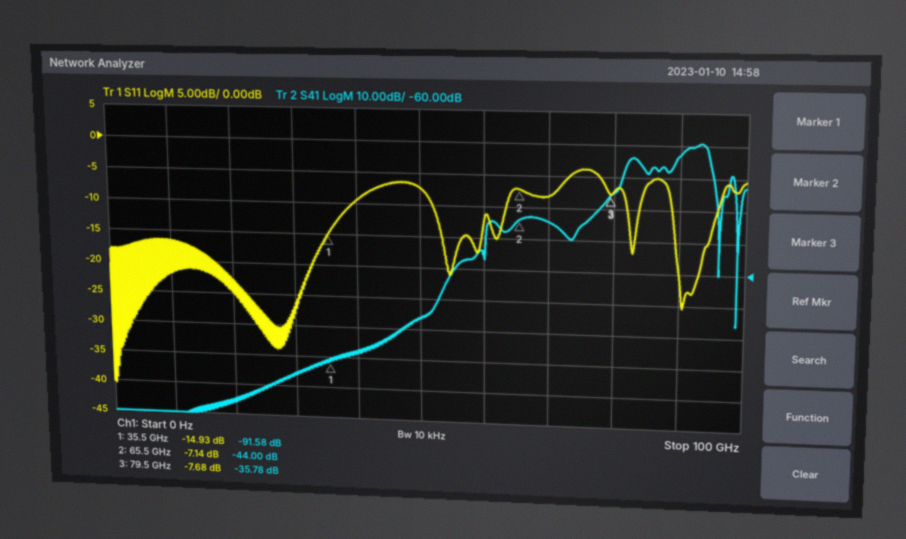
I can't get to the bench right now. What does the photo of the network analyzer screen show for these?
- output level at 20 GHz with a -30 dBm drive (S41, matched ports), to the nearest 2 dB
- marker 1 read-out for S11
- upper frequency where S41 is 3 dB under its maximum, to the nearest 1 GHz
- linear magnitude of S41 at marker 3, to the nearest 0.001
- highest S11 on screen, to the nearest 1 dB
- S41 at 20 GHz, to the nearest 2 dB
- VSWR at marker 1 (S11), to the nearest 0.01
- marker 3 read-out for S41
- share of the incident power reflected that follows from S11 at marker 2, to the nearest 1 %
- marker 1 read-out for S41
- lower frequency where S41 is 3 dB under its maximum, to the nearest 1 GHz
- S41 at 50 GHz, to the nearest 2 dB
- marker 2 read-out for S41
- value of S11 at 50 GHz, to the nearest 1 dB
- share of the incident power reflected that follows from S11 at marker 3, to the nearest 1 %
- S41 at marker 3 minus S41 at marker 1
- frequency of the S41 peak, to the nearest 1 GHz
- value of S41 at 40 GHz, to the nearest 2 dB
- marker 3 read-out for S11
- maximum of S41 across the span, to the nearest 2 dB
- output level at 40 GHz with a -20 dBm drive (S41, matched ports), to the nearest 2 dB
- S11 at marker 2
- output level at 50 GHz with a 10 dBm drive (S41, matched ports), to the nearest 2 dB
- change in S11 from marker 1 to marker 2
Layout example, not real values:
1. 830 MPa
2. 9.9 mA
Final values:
1. -136 dBm
2. -14.93 dB
3. 94 GHz
4. 0.016
5. -4 dB
6. -106 dB
7. 1.44
8. -35.78 dB
9. 19 %
10. -91.58 dB
11. 90 GHz
12. -76 dB
13. -44.00 dB
14. -7 dB
15. 17 %
16. 55.80 dB
17. 93 GHz
18. -88 dB
19. -7.68 dB
20. -20 dB
21. -108 dBm
22. -7.14 dB
23. -66 dBm
24. 7.79 dB
